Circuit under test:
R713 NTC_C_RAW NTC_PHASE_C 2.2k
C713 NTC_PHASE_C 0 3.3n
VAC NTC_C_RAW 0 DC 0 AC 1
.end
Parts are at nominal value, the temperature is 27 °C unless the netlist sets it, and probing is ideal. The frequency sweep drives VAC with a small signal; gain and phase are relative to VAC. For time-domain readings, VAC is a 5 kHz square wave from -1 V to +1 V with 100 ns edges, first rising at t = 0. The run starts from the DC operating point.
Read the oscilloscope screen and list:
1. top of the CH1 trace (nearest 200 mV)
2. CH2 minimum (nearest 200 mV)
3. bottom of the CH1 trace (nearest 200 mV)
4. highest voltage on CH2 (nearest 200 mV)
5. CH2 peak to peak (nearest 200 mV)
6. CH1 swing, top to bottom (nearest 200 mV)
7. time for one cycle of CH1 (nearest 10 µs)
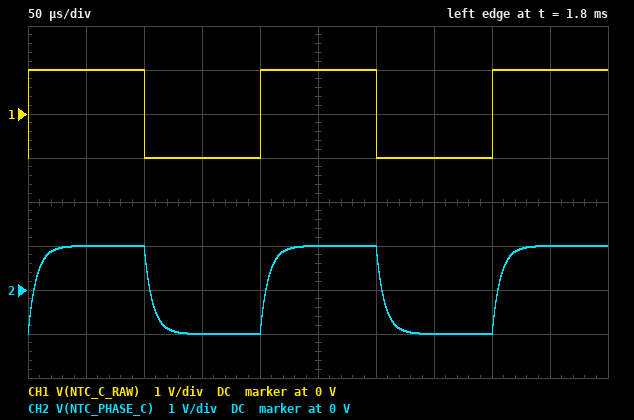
1.0 V
-1.0 V
-1.0 V
1.0 V
2.0 V
2.0 V
200 µs
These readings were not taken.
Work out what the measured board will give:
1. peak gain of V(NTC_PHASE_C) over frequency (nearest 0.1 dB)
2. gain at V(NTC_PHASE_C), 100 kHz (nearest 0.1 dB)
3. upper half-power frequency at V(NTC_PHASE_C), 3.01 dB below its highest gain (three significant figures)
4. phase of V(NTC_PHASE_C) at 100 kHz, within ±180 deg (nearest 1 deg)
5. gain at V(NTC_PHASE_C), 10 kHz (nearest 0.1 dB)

0 dB
-13.4 dB
21.9 kHz
-78 deg
-0.8 dB
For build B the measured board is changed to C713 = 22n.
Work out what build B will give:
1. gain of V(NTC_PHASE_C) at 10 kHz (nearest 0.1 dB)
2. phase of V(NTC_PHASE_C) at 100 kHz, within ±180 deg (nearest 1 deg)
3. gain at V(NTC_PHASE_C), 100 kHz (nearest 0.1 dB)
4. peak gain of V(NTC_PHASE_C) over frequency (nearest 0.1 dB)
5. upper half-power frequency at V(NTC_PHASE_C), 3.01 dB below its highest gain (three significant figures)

-10.1 dB
-88 deg
-29.7 dB
0 dB
3.29 kHz
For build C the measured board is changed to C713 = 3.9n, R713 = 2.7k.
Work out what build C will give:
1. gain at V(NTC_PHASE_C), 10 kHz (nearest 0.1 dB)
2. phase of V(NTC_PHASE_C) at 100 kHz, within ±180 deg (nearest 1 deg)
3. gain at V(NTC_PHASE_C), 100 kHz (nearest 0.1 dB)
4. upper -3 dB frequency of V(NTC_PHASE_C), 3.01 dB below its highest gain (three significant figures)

-1.6 dB
-81 deg
-16.5 dB
15.1 kHz
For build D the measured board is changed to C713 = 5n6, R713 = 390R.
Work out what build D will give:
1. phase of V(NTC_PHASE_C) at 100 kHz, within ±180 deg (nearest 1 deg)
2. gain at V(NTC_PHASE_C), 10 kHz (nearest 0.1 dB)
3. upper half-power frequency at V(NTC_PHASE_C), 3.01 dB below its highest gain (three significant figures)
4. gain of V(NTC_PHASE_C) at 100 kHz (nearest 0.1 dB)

-54 deg
-0.1 dB
72.9 kHz
-4.6 dB
